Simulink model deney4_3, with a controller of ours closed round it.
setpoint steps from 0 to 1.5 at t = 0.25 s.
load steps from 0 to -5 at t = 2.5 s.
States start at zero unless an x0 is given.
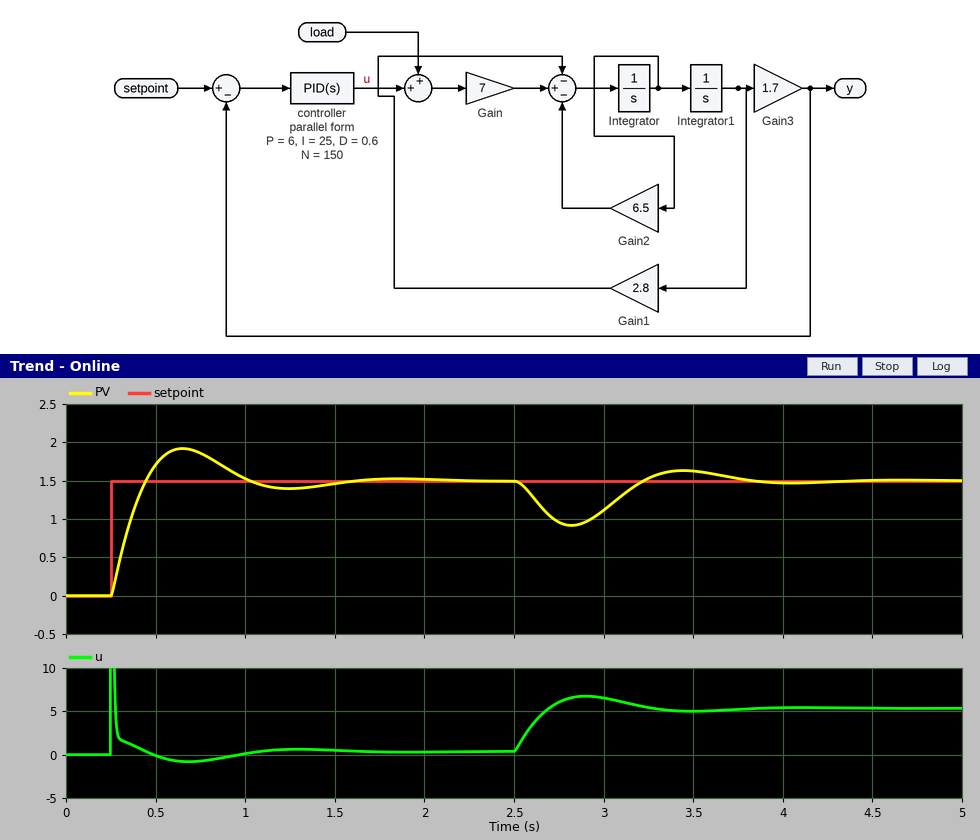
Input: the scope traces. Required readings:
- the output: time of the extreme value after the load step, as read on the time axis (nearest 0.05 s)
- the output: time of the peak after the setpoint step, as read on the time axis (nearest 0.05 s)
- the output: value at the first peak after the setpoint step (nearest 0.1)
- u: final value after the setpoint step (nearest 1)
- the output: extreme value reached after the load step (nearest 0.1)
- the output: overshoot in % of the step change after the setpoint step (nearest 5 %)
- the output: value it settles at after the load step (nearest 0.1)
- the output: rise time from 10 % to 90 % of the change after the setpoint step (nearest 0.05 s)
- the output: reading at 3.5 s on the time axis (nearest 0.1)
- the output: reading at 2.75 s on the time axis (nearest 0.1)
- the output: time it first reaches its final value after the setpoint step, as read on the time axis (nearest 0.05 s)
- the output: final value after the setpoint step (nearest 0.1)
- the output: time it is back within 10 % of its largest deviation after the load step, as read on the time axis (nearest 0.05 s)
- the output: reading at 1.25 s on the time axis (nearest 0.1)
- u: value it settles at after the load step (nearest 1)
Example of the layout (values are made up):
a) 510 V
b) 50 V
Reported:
a) 2.80 s
b) 0.65 s
c) 1.9
d) 0
e) 0.9
f) 30 %
g) 1.5
h) 0.15 s
i) 1.6
j) 1.0
k) 0.45 s
l) 1.5
m) 3.70 s
n) 1.4
o) 5
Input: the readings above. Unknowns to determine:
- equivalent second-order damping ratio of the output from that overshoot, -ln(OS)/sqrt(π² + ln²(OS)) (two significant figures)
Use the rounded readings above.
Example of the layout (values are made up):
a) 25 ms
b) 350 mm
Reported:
a) 0.36
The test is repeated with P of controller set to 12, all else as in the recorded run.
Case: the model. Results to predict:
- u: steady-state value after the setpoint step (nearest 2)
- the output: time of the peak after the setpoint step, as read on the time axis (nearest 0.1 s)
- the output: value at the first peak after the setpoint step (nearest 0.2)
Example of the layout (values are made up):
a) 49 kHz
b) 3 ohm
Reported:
a) 0
b) 0.5 s
c) 1.8
